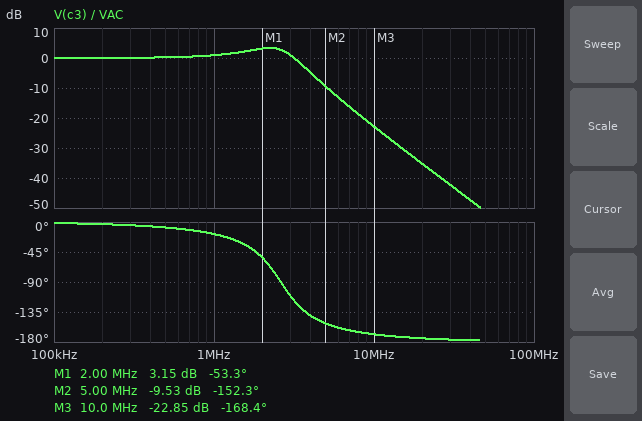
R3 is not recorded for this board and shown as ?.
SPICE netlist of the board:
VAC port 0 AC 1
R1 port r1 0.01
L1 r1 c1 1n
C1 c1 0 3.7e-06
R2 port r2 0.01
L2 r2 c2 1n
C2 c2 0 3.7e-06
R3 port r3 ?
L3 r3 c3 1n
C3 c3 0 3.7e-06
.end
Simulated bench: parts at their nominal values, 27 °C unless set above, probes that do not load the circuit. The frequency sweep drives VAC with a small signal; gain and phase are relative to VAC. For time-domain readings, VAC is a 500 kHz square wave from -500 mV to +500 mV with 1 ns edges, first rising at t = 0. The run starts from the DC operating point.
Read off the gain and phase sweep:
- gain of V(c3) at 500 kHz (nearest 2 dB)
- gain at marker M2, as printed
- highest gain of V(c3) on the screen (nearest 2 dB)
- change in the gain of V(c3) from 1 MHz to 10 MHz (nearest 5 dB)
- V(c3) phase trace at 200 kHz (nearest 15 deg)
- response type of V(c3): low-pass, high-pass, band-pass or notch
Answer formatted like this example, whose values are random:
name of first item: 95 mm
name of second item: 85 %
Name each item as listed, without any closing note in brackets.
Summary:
gain of V(c3) at 500 kHz: 0 dB
gain at marker M2, as printed: -9.53 dB
highest gain of V(c3) on the screen: 4 dB
change in the gain of V(c3) from 1 MHz to 10 MHz: -25 dB
V(c3) phase trace at 200 kHz: 0 deg
response type of V(c3): low-pass, high-pass, band-pass or notch: low-pass
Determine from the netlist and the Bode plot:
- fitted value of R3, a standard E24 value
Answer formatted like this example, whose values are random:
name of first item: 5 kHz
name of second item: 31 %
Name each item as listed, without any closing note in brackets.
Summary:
fitted value of R3, a standard E24 value: 0.012 Ω
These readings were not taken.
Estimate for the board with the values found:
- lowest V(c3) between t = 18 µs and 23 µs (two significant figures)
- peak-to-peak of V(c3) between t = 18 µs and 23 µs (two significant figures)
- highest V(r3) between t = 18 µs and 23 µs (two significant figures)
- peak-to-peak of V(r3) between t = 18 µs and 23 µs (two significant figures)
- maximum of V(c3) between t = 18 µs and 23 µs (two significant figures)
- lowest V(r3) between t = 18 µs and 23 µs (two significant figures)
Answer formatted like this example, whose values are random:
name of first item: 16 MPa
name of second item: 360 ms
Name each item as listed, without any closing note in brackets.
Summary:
lowest V(c3) between t = 18 µs and 23 µs: -790 mV
peak-to-peak of V(c3) between t = 18 µs and 23 µs: 1.6 V
highest V(r3) between t = 18 µs and 23 µs: 630 mV
peak-to-peak of V(r3) between t = 18 µs and 23 µs: 1.3 V
maximum of V(c3) between t = 18 µs and 23 µs: 790 mV
lowest V(r3) between t = 18 µs and 23 µs: -630 mV
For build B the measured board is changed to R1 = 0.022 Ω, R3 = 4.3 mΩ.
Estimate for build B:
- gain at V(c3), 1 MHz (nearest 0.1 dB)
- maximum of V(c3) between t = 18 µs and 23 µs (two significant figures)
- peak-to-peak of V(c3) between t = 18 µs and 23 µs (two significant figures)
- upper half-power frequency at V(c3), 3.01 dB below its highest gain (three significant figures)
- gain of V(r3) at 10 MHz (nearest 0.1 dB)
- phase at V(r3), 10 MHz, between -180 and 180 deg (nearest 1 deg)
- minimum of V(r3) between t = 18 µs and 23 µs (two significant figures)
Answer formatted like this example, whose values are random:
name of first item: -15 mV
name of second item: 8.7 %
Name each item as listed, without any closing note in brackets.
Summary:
gain at V(c3), 1 MHz: 1.3 dB
maximum of V(c3) between t = 18 µs and 23 µs: 1.2 V
peak-to-peak of V(c3) between t = 18 µs and 23 µs: 2.5 V
upper half-power frequency at V(c3), 3.01 dB below its highest gain: 2.90 MHz
gain of V(r3) at 10 MHz: 0 dB
phase at V(r3), 10 MHz, between -180 and 180 deg: 4 deg
minimum of V(r3) between t = 18 µs and 23 µs: -660 mV
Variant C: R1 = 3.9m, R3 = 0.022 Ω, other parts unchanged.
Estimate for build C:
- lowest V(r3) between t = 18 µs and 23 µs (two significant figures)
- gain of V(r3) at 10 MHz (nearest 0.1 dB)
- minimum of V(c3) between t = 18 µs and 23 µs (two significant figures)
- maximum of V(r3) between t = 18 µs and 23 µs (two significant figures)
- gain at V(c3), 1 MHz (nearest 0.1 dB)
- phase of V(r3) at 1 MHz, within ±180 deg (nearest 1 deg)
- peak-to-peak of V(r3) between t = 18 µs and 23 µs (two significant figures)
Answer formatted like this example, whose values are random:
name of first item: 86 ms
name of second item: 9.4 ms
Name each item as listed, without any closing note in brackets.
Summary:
lowest V(r3) between t = 18 µs and 23 µs: -540 mV
gain of V(r3) at 10 MHz: -0.6 dB
minimum of V(c3) between t = 18 µs and 23 µs: -560 mV
maximum of V(r3) between t = 18 µs and 23 µs: 540 mV
gain at V(c3), 1 MHz: 0 dB
phase of V(r3) at 1 MHz, within ±180 deg: -31 deg
peak-to-peak of V(r3) between t = 18 µs and 23 µs: 1.1 V
